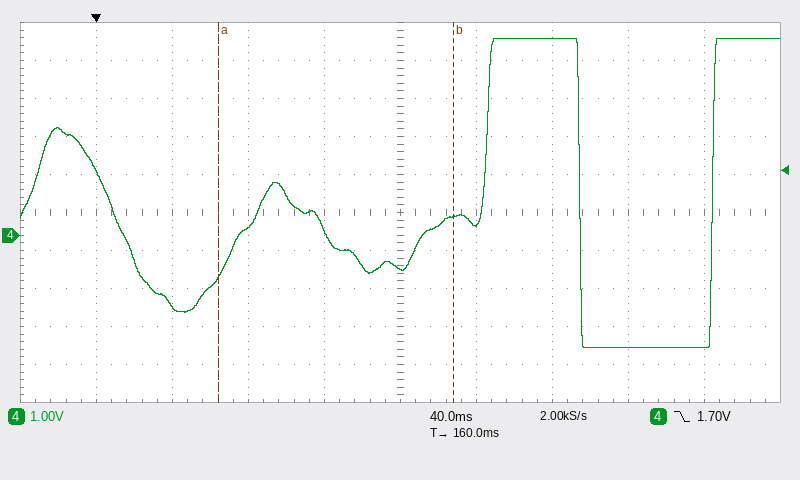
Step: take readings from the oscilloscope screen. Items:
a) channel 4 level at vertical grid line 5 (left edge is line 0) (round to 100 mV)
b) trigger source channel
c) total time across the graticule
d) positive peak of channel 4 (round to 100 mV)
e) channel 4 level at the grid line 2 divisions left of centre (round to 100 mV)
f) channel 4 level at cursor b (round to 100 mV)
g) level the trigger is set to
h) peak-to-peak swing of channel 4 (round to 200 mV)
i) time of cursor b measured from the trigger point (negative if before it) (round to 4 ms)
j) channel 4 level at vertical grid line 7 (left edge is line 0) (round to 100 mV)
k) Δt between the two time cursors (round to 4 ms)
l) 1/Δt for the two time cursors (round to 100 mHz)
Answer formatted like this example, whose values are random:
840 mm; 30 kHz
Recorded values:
-900 mV; channel 4; 400 ms; 5.2 V; 200 mV; 500 mV; 1.70 V; 8.2 V; +188 ms; 5.2 V; 124 ms; 8.1 Hz
